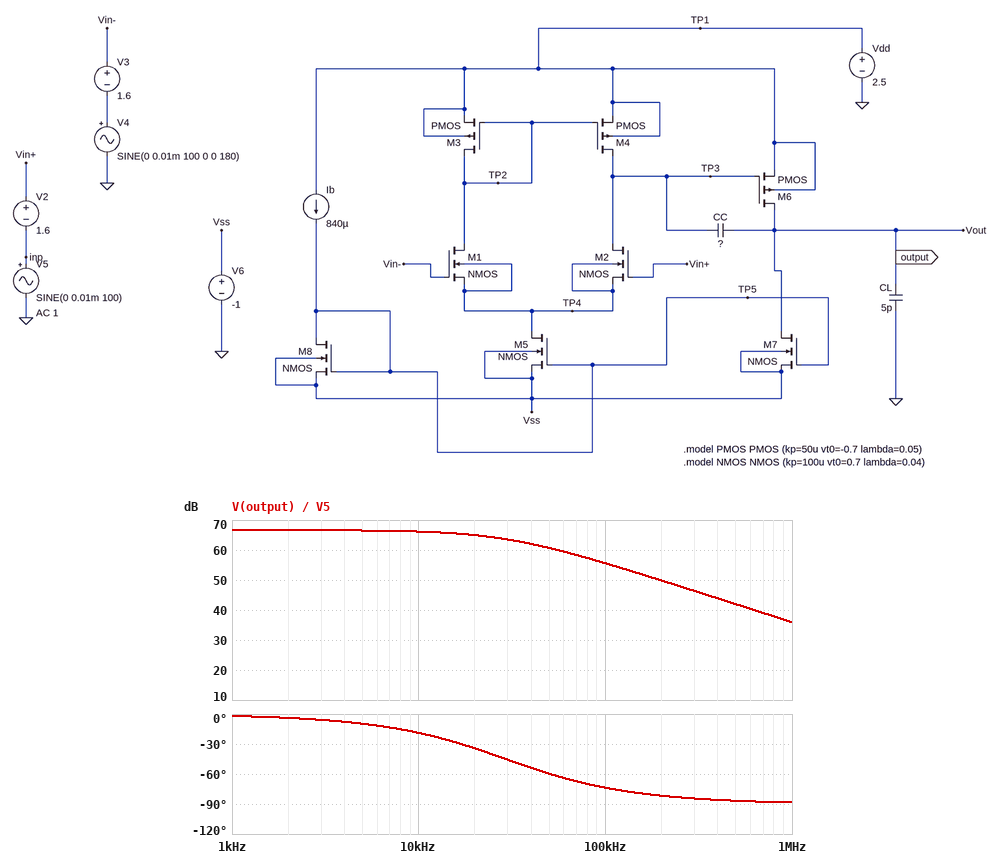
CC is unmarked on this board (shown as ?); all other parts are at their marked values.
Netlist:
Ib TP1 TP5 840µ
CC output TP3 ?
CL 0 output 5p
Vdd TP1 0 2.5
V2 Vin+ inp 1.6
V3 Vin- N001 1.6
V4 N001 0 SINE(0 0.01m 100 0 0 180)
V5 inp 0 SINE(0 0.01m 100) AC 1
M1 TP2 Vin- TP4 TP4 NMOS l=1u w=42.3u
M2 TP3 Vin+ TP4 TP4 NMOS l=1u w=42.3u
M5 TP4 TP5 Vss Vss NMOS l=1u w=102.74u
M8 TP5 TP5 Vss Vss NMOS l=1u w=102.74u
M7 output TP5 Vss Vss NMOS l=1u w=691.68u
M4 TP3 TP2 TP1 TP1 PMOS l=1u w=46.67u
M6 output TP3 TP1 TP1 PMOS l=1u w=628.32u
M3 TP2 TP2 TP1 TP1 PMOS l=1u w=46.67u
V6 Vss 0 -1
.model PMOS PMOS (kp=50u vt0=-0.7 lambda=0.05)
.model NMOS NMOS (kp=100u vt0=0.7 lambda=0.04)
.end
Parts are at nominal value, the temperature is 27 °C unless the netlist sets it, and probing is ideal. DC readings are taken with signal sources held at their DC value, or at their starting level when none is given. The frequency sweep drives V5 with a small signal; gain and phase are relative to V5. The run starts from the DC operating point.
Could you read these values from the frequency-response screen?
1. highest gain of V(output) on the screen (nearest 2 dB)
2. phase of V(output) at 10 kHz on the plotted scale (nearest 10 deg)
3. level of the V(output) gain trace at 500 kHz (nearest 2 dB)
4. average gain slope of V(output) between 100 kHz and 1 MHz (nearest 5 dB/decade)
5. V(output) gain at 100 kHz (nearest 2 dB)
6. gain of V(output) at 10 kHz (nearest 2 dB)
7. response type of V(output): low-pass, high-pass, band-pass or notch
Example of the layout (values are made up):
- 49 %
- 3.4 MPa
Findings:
- 66 dB
- -20 deg
- 42 dB
- -20 dB/decade
- 56 dB
- 66 dB
- low-pass
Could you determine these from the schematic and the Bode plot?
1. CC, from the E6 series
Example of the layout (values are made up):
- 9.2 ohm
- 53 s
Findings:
- 4.7 pF
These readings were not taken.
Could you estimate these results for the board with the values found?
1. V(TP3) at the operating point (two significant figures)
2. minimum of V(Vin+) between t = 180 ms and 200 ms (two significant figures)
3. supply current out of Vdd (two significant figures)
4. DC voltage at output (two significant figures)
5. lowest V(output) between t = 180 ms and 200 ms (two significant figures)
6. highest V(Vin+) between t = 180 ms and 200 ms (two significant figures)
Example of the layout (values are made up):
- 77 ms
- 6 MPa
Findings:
- 1.2 V
- 1.6 V
- 7.5 mA
- 880 mV
- 830 mV
- 1.6 V
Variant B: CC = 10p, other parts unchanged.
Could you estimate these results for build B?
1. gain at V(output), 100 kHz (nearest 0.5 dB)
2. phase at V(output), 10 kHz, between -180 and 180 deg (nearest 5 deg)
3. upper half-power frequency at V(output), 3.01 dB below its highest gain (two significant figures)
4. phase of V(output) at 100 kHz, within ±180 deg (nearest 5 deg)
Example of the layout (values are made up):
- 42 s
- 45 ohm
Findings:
- 49.5 dB
- -35 deg
- 14 kHz
- -80 deg
